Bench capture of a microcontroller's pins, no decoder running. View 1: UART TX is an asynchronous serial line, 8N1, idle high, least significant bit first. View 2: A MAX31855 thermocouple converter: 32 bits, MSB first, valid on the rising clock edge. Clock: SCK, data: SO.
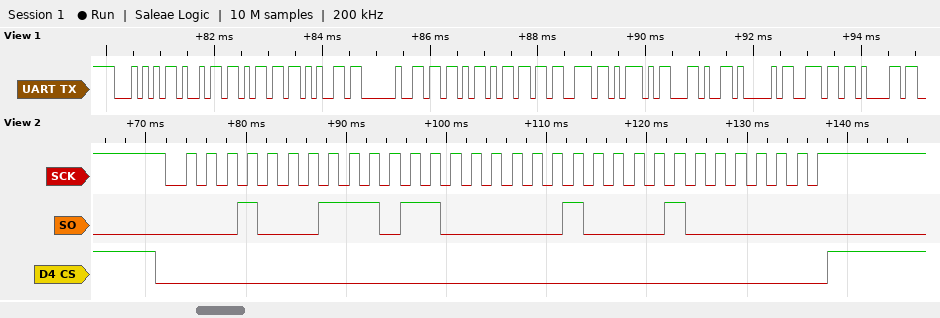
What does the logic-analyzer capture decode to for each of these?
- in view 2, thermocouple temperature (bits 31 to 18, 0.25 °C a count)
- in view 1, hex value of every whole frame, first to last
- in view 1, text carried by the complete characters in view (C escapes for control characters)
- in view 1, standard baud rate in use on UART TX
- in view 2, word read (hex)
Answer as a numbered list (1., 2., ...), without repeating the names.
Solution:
1. 285.50 °C
2. 54 69 6D 65 20 5B 6D 73 5D 2C 41 6E 61
3. "Time [ms],Ana"
4. 9600 baud
5. 0x11D81080
